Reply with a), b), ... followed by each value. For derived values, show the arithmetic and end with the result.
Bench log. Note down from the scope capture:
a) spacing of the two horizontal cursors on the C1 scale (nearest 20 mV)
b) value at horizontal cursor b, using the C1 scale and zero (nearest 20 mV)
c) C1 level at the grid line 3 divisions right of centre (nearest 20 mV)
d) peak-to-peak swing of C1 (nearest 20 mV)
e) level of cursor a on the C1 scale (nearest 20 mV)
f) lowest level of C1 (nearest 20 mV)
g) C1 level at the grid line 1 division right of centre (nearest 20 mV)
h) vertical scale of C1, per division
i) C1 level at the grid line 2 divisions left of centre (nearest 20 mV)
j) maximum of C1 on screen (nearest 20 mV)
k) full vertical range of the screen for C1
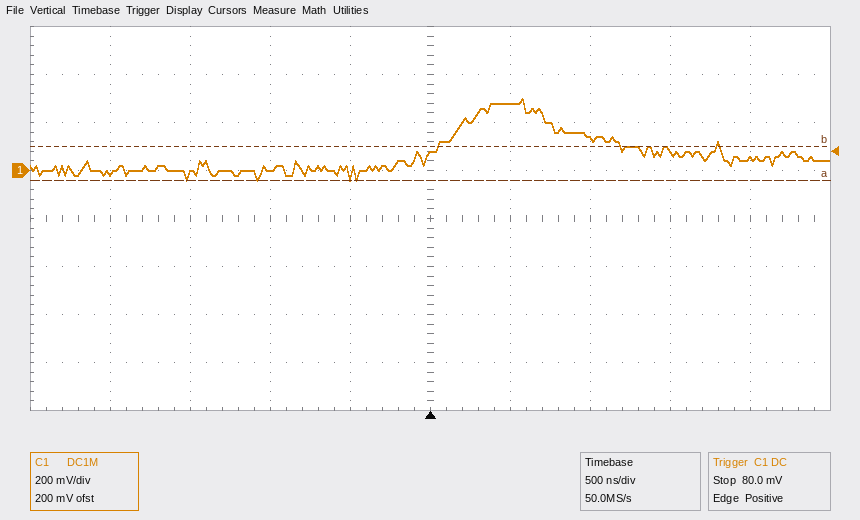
a) 140 mV
b) 100 mV
c) 80 mV
d) 300 mV − (-40 mV) = 340 mV
e) -40 mV
f) -40 mV
g) 280 mV
h) 200 mV
i) 0 mV
j) 300 mV
k) 1.6 V
